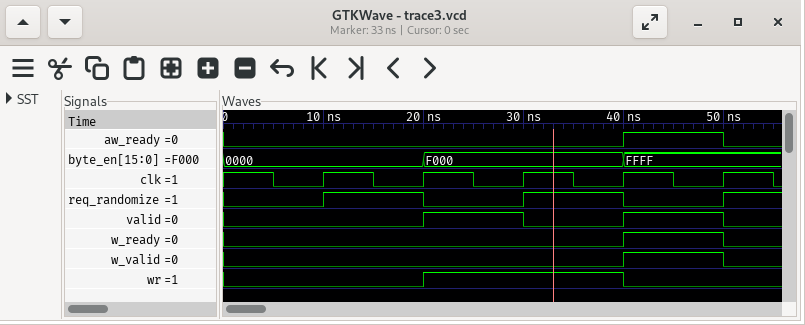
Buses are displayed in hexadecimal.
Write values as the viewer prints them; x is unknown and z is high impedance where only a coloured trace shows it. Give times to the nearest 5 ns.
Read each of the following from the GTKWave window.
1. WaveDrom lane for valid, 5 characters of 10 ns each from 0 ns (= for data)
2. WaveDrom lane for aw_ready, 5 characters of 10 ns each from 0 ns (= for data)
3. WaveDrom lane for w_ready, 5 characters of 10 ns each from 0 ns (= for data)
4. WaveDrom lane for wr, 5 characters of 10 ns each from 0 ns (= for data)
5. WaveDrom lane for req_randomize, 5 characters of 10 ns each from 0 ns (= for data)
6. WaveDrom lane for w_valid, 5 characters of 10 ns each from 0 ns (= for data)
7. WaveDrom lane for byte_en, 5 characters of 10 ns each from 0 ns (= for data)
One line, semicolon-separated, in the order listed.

{name: 'valid', wave: '0.101'}; {name: 'aw_ready', wave: '0...1'}; {name: 'w_ready', wave: '0...1'}; {name: 'wr', wave: '0.1.0'}; {name: 'req_randomize', wave: '01010'}; {name: 'w_valid', wave: '0...1'}; {name: 'byte_en', wave: '=.=.=', data: '0000 F000 FFFF'}
